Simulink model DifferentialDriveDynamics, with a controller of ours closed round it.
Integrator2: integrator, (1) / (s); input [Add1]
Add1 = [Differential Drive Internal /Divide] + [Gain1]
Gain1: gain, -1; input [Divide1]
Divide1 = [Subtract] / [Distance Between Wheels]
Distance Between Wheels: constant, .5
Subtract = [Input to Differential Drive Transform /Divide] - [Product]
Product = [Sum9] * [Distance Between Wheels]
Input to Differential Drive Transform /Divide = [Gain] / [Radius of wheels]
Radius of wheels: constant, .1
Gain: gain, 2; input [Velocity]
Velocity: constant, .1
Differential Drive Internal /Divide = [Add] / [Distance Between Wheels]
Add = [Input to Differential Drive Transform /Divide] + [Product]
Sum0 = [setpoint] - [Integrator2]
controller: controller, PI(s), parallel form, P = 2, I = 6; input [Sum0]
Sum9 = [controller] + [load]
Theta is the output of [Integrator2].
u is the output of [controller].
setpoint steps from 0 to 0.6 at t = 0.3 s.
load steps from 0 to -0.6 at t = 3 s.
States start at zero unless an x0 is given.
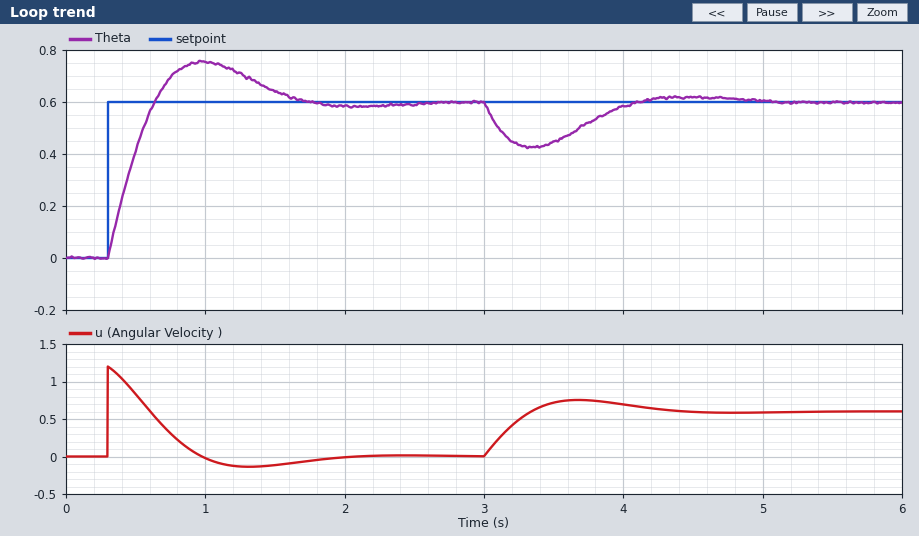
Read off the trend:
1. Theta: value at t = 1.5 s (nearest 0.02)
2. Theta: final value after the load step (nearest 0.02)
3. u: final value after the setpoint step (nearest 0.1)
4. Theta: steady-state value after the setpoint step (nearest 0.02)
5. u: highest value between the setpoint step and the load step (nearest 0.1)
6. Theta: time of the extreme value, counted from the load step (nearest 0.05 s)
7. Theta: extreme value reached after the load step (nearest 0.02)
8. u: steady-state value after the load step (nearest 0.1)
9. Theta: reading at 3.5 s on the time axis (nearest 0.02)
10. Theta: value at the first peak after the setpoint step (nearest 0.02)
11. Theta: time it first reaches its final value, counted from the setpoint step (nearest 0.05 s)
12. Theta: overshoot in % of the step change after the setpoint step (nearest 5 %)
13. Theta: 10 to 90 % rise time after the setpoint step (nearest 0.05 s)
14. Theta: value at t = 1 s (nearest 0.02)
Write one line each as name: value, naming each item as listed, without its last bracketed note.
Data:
Theta: value at t = 1.5 s: 0.64
Theta: final value after the load step: 0.60
u: final value after the setpoint step: 0.0
Theta: steady-state value after the setpoint step: 0.60
u: highest value between the setpoint step and the load step: 1.2
Theta: time of the extreme value, counted from the load step: 0.35 s
Theta: extreme value reached after the load step: 0.42
u: steady-state value after the load step: 0.6
Theta: reading at 3.5 s on the time axis: 0.44
Theta: value at the first peak after the setpoint step: 0.76
Theta: time it first reaches its final value, counted from the setpoint step: 0.35 s
Theta: overshoot in % of the step change after the setpoint step: 25 %
Theta: 10 to 90 % rise time after the setpoint step: 0.25 s
Theta: value at t = 1 s: 0.76
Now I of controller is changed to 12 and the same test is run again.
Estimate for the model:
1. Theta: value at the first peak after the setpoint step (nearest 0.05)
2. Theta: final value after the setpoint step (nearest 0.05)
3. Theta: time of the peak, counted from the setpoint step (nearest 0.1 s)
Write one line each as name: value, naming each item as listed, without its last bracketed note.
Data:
Theta: value at the first peak after the setpoint step: 0.80
Theta: final value after the setpoint step: 0.60
Theta: time of the peak, counted from the setpoint step: 0.5 s
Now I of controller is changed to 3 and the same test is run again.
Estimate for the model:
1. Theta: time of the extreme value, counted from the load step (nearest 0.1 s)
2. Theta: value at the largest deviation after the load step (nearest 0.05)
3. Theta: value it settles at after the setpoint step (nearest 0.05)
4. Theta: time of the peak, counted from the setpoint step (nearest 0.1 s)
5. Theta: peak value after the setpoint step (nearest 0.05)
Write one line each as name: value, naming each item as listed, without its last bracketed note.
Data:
Theta: time of the extreme value, counted from the load step: 0.4 s
Theta: value at the largest deviation after the load step: 0.40
Theta: value it settles at after the setpoint step: 0.60
Theta: time of the peak, counted from the setpoint step: 0.9 s
Theta: peak value after the setpoint step: 0.70
